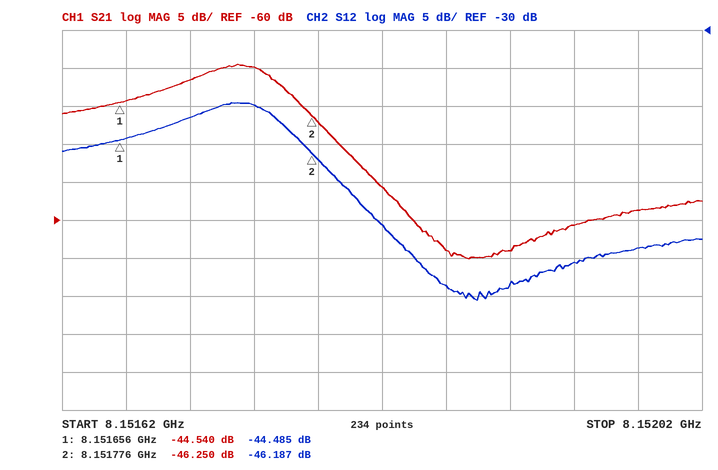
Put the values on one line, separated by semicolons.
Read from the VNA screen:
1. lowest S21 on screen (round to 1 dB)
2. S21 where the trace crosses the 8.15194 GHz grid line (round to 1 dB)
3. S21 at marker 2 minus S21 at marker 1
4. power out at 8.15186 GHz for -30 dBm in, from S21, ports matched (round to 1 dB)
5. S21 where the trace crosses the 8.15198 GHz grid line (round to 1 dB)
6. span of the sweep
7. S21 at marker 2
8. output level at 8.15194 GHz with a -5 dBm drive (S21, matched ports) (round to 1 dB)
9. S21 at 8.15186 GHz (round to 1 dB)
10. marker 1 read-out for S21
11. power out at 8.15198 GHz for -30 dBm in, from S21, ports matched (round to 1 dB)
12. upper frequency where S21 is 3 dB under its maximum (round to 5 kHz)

-65 dB; -61 dB; -1.710 dB; -94 dBm; -59 dB; 400 kHz; -46.250 dB; -66 dBm; -64 dB; -44.540 dB; -89 dBm; 8.151760 GHz
